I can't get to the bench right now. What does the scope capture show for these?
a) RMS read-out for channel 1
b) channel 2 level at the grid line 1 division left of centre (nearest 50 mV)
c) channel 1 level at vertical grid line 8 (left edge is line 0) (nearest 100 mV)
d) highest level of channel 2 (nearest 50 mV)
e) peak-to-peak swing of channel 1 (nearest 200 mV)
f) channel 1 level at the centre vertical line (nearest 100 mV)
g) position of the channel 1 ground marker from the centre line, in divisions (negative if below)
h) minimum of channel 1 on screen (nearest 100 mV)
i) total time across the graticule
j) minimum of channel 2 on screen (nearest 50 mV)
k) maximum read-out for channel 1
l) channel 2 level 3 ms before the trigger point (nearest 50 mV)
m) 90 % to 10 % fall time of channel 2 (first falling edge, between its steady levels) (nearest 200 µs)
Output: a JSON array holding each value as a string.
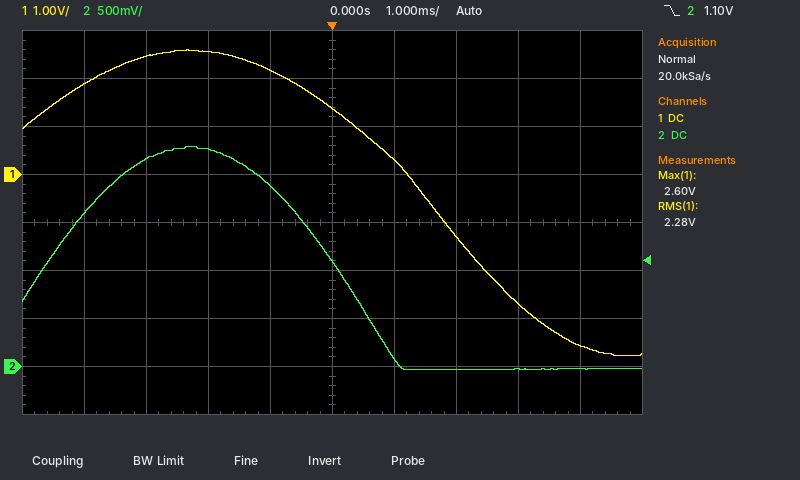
["2.28 V", "1.90 V", "-2.7 V", "2.30 V", "6.4 V", "1.4 V", "+1.0 div", "-3.8 V", "10 ms", "-50 mV", "2.60 V", "2.15 V", "2.2 ms"]
